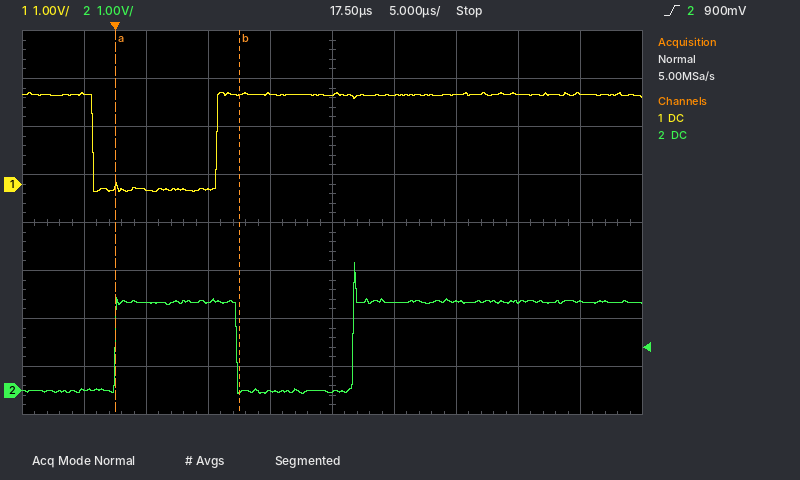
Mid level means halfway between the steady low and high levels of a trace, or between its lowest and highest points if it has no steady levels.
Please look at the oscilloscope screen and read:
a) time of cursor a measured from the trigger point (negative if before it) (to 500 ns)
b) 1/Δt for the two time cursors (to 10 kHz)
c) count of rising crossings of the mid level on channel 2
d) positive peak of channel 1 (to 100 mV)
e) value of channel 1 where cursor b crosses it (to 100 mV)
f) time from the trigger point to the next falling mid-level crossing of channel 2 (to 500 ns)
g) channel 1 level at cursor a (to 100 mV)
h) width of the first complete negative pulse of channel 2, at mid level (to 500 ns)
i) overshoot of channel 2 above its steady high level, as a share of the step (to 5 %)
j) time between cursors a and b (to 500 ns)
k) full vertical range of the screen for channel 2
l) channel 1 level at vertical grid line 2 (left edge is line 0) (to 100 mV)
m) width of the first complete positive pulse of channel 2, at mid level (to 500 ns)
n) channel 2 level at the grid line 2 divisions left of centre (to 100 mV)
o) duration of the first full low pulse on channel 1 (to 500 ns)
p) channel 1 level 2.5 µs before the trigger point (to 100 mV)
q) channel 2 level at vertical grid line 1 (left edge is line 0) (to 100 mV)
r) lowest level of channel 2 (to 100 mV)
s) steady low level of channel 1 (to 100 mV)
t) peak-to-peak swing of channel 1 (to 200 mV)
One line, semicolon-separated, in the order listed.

0.0 µs; 100 kHz; 2; 1.9 V; 1.9 V; 10.0 µs; -100 mV; 9.5 µs; 45 %; 10.0 µs; 8 V; -100 mV; 10.0 µs; 1.8 V; 10.0 µs; 1.9 V; 0.0 V; -100 mV; -100 mV; 2.0 V
